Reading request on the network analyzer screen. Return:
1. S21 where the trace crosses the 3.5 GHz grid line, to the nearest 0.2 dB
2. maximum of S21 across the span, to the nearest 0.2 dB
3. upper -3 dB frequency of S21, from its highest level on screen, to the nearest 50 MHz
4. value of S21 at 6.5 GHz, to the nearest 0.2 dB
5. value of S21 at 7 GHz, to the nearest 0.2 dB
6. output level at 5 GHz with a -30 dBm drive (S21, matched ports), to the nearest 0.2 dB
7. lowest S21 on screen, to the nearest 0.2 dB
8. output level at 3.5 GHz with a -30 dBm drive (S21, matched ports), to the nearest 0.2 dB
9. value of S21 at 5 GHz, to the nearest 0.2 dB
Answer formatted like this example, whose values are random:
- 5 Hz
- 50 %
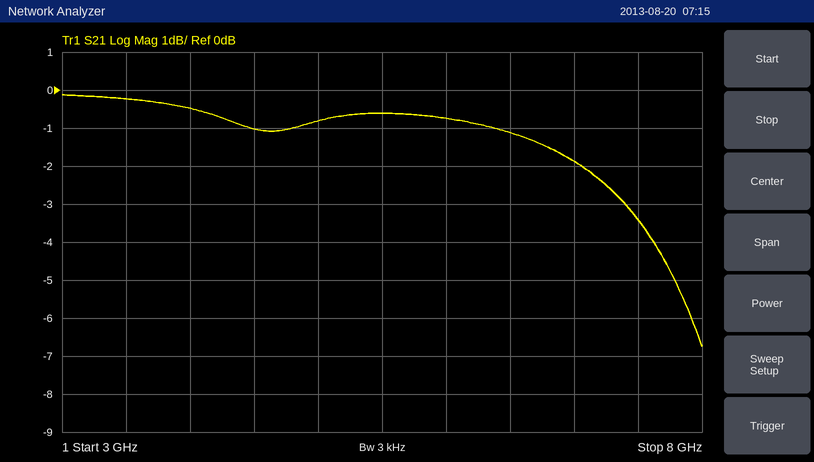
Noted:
- -0.2 dB
- -0.2 dB
- 7.45 GHz
- -1.2 dB
- -1.8 dB
- -30.8 dBm
- -6.8 dB
- -30.2 dBm
- -0.8 dB
